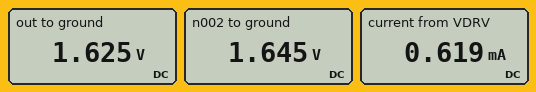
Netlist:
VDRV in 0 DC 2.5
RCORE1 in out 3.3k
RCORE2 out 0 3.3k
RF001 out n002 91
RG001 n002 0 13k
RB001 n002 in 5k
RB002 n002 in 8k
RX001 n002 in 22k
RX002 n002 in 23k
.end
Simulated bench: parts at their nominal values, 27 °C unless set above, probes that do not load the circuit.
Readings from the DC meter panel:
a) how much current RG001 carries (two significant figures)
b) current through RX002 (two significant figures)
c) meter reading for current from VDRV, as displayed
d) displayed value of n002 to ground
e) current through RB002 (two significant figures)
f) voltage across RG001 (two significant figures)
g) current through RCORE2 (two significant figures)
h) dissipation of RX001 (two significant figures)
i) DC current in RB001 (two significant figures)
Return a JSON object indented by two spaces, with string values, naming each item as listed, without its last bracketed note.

{
  "how much current RG001 carries": "130 µA",
  "current through RX002": "37 µA",
  "meter reading for current from VDRV, as displayed": "0.619 mA",
  "displayed value of n002 to ground": "1.645 V",
  "current through RB002": "110 µA",
  "voltage across RG001": "1.6 V",
  "current through RCORE2": "490 µA",
  "dissipation of RX001": "33 µW",
  "DC current in RB001": "170 µA"
}
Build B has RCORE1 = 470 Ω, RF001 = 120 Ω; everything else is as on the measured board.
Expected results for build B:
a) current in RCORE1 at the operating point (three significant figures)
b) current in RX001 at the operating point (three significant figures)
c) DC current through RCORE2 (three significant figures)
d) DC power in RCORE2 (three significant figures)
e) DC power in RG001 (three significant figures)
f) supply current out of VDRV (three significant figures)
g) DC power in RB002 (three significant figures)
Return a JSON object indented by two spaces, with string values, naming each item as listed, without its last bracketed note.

{
  "current in RCORE1 at the operating point": "690 µA",
  "current in RX001 at the operating point": "14.9 µA",
  "DC current through RCORE2": "659 µA",
  "DC power in RCORE2": "1.43 mW",
  "DC power in RG001": "363 µW",
  "supply current out of VDRV": "826 µA",
  "DC power in RB002": "13.5 µW"
}
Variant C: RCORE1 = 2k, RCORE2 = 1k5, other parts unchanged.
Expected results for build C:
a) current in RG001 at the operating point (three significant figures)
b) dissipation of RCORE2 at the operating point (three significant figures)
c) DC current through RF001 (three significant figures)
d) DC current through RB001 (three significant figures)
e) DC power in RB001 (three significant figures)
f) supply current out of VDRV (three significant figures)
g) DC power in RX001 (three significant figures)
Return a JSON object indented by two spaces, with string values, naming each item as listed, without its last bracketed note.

{
  "current in RG001 at the operating point": "108 µA",
  "dissipation of RCORE2 at the operating point": "1.25 mW",
  "DC current through RF001": "347 µA",
  "DC current through RB001": "220 µA",
  "DC power in RB001": "242 µW",
  "supply current out of VDRV": "1.02 mA",
  "DC power in RX001": "54.9 µW"
}
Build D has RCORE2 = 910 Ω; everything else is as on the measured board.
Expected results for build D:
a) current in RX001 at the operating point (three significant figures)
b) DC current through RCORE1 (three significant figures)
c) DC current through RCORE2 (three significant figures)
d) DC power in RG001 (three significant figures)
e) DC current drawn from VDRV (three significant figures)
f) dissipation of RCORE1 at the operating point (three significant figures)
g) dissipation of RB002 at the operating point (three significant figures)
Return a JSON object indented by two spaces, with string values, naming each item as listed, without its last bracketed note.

{
  "current in RX001 at the operating point": "68.9 µA",
  "DC current through RCORE1": "475 µA",
  "DC current through RCORE2": "1.03 mA",
  "DC power in RG001": "74.5 µW",
  "DC current drawn from VDRV": "1.10 mA",
  "dissipation of RCORE1 at the operating point": "743 µW",
  "dissipation of RB002 at the operating point": "287 µW"
}
